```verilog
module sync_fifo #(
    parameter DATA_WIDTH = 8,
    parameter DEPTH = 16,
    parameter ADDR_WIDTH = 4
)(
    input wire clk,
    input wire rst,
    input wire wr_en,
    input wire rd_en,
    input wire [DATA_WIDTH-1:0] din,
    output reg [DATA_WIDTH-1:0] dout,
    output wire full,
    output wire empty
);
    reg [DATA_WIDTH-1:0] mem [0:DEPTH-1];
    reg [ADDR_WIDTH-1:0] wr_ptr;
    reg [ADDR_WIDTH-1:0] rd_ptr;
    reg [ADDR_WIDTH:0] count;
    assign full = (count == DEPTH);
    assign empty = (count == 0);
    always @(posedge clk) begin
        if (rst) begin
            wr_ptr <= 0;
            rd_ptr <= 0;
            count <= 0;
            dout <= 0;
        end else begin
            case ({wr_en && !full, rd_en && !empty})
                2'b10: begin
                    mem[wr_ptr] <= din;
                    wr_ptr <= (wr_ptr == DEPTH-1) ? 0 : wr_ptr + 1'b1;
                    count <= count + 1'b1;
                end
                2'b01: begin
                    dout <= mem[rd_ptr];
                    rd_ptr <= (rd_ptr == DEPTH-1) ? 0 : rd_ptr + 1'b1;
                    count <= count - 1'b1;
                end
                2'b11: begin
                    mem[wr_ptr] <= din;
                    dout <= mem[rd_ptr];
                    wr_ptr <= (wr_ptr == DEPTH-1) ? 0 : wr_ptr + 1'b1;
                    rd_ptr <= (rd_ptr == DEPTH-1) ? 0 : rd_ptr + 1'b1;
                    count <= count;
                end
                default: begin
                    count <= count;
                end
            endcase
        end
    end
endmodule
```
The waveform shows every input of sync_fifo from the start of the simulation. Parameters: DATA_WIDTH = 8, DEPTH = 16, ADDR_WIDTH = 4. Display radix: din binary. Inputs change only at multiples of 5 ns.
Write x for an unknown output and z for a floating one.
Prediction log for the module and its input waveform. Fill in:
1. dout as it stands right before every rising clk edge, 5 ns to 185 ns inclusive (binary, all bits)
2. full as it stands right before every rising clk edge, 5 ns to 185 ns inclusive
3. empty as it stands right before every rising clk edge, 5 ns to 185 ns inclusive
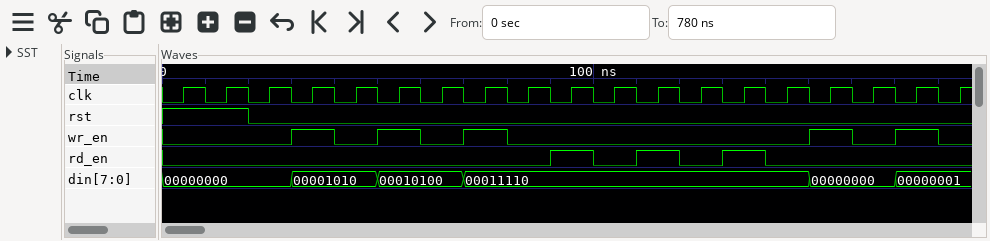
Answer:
x, 00000000, 00000000, 00000000, 00000000, 00000000, 00000000, 00000000, 00000000, 00000000, 00001010, 00001010, 00010100, 00010100, 00011110, 00011110, 00011110, 00011110, 00011110
x 0 0 0 0 0 0 0 0 0 0 0 0 0 0 0 0 0 0
x 1 1 1 0 0 0 0 0 0 0 0 0 0 1 1 0 0 0
